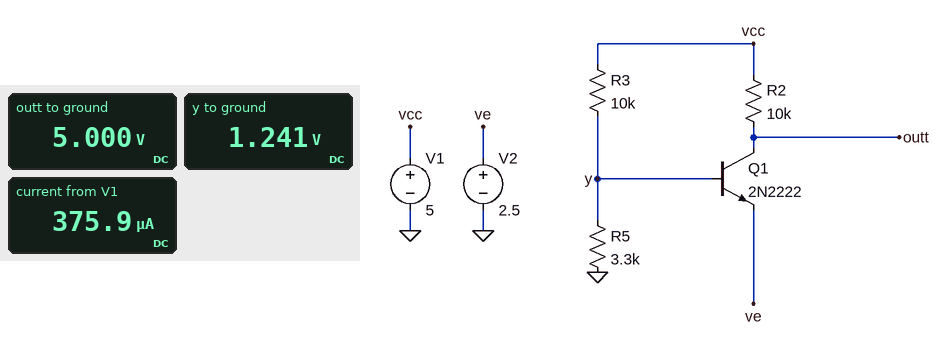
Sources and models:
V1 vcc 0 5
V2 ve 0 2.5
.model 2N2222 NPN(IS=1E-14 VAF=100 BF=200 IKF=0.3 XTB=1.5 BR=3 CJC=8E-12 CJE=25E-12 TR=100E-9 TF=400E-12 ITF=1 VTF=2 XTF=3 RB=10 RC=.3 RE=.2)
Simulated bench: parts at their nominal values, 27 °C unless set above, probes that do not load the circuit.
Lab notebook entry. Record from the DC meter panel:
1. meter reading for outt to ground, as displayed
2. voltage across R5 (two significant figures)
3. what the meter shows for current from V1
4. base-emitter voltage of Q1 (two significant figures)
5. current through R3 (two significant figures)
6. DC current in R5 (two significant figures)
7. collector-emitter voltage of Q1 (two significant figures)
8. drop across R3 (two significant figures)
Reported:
5.000 V
1.2 V
375.9 µA
-1.3 V
380 µA
380 µA
2.5 V
3.8 V
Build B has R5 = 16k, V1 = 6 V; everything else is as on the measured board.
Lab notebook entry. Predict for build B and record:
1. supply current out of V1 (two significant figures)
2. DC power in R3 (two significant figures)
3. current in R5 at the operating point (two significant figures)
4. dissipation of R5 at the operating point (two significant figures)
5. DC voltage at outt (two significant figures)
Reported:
630 µA
810 µW
200 µA
620 µW
2.5 V
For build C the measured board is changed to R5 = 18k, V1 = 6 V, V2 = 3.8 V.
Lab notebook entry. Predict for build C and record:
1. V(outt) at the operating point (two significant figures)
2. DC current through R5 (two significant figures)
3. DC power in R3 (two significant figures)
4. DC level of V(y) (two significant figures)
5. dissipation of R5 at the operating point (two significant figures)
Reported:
6.0 V
210 µA
460 µW
3.9 V
830 µW
